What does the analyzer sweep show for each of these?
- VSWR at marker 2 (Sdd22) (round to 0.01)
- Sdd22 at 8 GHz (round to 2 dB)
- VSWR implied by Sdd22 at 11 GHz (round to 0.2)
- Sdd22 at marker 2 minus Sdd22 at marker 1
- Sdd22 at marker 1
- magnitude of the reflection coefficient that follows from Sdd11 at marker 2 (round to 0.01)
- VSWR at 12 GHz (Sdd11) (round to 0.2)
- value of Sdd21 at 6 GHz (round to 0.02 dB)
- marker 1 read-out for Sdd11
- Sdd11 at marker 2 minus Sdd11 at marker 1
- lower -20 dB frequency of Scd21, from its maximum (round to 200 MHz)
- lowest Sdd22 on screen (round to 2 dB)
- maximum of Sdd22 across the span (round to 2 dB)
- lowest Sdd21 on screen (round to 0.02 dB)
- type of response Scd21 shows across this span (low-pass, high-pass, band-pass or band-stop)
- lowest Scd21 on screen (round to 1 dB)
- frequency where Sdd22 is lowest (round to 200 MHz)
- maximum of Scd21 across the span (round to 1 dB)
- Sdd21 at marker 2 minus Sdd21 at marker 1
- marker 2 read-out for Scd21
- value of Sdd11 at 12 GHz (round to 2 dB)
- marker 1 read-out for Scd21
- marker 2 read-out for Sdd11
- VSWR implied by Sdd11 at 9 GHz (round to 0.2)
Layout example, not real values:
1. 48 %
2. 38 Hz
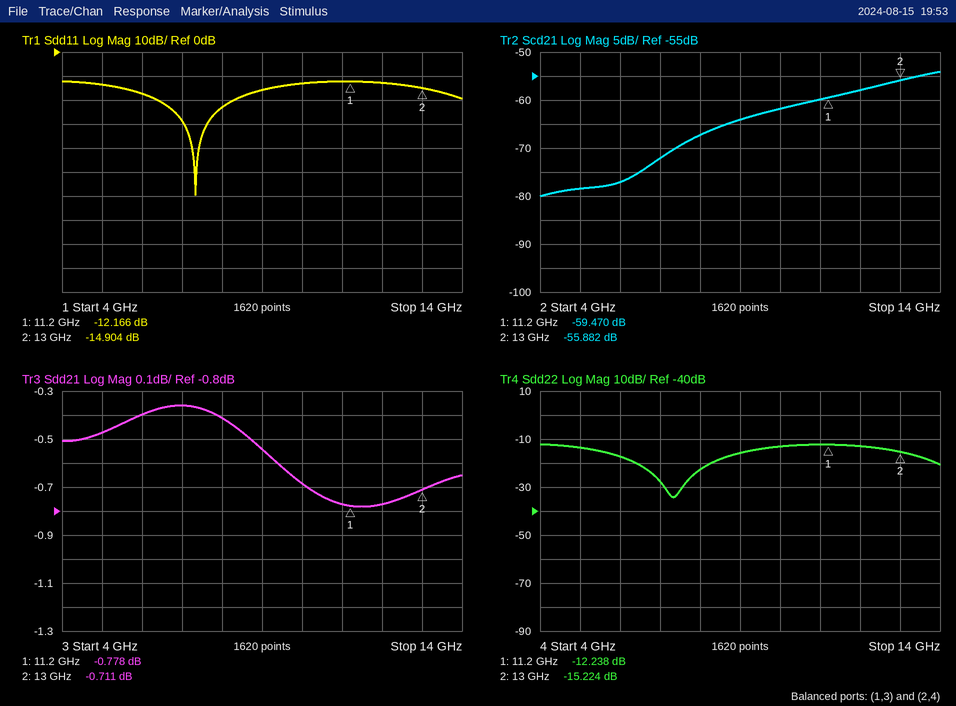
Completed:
1. 1.42
2. -22 dB
3. 1.6
4. -2.986 dB
5. -12.238 dB
6. 0.18
7. 1.6
8. -0.40 dB
9. -12.166 dB
10. -2.738 dB
11. 6.6 GHz
12. -34 dB
13. -12 dB
14. -0.78 dB
15. high-pass
16. -80 dB
17. 7.4 GHz
18. -54 dB
19. 0.067 dB
20. -55.882 dB
21. -12 dB
22. -59.470 dB
23. -14.904 dB
24. 1.4
